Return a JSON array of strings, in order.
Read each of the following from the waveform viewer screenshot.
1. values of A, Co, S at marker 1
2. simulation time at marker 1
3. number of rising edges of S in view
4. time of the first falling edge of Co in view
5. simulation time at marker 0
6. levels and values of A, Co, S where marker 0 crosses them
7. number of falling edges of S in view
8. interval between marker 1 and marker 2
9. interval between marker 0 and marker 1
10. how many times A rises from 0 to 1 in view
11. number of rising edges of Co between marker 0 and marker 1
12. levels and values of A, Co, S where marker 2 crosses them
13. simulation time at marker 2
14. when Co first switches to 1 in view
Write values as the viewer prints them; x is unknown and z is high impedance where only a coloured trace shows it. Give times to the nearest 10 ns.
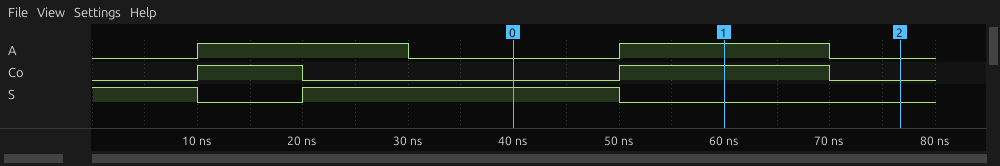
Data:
["A=1, Co=1, S=0", "60 ns", "1", "20 ns", "40 ns", "A=0, Co=0, S=1", "2", "20 ns", "20 ns", "2", "1", "A=0, Co=0, S=0", "80 ns", "10 ns"]
